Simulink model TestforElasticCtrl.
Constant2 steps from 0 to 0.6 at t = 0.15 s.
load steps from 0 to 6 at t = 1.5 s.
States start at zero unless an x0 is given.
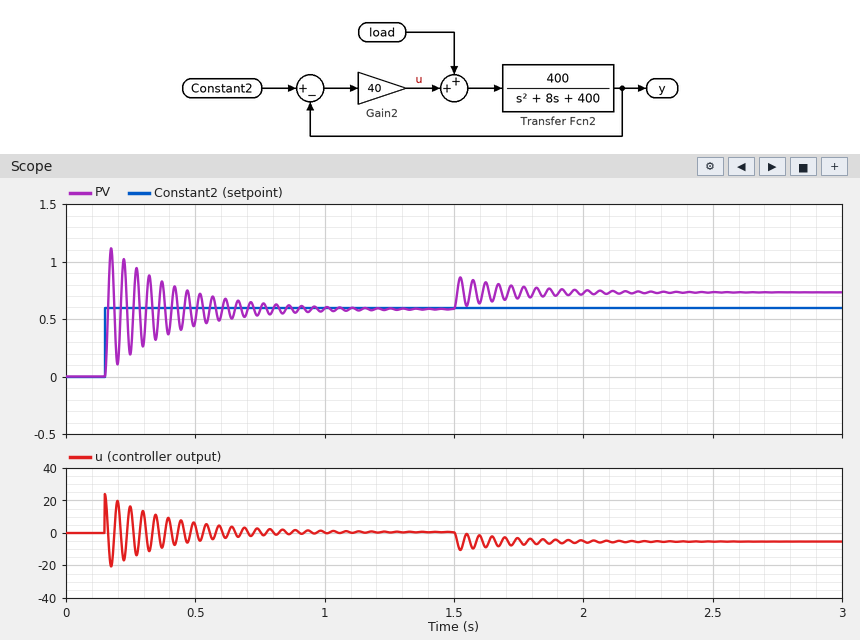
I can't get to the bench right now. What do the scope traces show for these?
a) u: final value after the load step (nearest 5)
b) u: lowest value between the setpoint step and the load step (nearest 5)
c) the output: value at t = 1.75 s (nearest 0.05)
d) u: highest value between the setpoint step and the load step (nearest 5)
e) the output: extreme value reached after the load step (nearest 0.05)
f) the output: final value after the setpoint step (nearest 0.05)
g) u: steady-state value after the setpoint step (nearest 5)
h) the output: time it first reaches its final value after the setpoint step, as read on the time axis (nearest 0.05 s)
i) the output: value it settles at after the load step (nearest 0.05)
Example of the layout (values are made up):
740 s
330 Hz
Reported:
-5
-20
0.70
25
0.85
0.60
0
0.15 s
0.75
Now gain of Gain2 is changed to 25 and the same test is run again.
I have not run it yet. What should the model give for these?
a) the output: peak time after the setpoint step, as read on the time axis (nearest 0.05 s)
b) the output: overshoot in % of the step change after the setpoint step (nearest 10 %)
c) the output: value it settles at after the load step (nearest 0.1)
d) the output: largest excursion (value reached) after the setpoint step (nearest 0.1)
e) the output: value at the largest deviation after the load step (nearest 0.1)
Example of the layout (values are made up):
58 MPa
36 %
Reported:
0.20 s
90 %
0.8
1.1
1.0
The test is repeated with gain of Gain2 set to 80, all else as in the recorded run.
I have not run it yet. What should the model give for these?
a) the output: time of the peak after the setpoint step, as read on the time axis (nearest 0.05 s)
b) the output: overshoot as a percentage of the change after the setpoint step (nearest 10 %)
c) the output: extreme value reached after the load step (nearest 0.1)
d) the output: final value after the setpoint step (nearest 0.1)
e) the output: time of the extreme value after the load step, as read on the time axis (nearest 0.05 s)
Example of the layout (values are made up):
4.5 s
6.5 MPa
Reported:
0.15 s
90 %
0.7
0.6
1.50 s
